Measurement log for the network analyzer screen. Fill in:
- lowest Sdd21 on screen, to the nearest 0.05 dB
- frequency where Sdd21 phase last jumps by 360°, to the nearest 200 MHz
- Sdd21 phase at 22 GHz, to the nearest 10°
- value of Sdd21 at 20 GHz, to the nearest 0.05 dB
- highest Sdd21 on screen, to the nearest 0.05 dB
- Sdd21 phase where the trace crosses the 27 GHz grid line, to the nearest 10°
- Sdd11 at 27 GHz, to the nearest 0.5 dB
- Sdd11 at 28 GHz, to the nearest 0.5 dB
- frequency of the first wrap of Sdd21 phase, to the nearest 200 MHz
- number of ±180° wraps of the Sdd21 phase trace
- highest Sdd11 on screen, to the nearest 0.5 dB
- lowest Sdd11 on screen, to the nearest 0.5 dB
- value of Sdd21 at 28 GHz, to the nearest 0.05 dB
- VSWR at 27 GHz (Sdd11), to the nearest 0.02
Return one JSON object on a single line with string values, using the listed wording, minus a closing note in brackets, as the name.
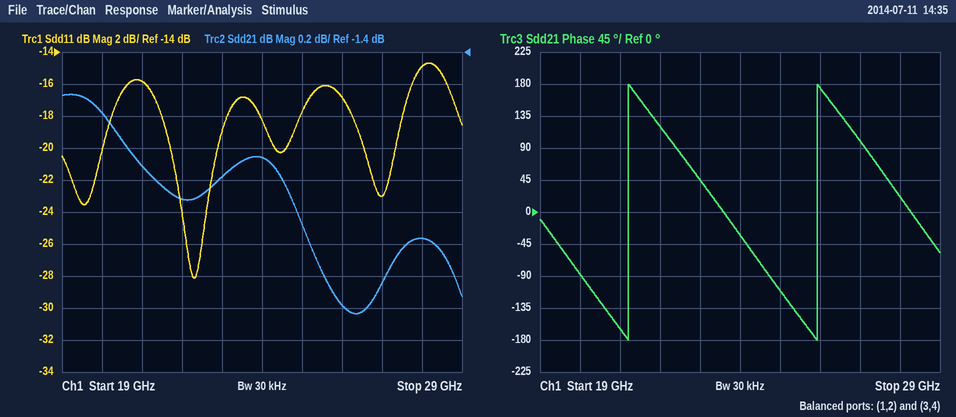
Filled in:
{"lowest Sdd21 on screen, to the nearest 0.05 dB": "-3.05 dB", "frequency where Sdd21 phase last jumps by 360°, to the nearest 200 MHz": "26.0 GHz", "Sdd21 phase at 22 GHz, to the nearest 10°": "120°", "value of Sdd21 at 20 GHz, to the nearest 0.05 dB": "-1.80 dB", "highest Sdd21 on screen, to the nearest 0.05 dB": "-1.65 dB", "Sdd21 phase where the trace crosses the 27 GHz grid line, to the nearest 10°": "100°", "Sdd11 at 27 GHz, to the nearest 0.5 dB": "-23.0 dB", "Sdd11 at 28 GHz, to the nearest 0.5 dB": "-15.0 dB", "frequency of the first wrap of Sdd21 phase, to the nearest 200 MHz": "21.2 GHz", "number of ±180° wraps of the Sdd21 phase trace": "2", "highest Sdd11 on screen, to the nearest 0.5 dB": "-14.5 dB", "lowest Sdd11 on screen, to the nearest 0.5 dB": "-28.0 dB", "value of Sdd21 at 28 GHz, to the nearest 0.05 dB": "-2.55 dB", "VSWR at 27 GHz (Sdd11), to the nearest 0.02": "1.16"}
